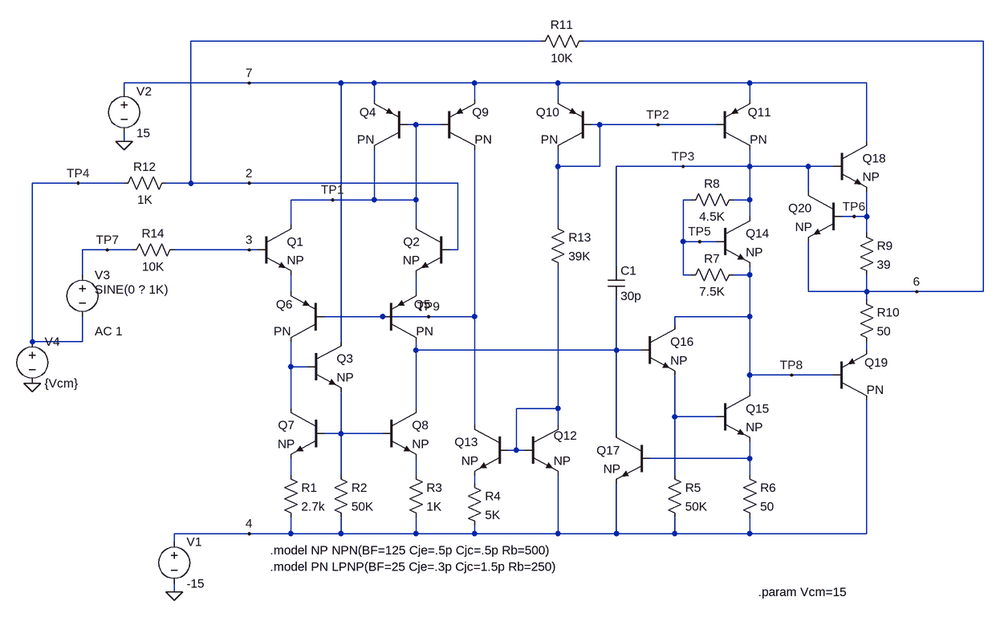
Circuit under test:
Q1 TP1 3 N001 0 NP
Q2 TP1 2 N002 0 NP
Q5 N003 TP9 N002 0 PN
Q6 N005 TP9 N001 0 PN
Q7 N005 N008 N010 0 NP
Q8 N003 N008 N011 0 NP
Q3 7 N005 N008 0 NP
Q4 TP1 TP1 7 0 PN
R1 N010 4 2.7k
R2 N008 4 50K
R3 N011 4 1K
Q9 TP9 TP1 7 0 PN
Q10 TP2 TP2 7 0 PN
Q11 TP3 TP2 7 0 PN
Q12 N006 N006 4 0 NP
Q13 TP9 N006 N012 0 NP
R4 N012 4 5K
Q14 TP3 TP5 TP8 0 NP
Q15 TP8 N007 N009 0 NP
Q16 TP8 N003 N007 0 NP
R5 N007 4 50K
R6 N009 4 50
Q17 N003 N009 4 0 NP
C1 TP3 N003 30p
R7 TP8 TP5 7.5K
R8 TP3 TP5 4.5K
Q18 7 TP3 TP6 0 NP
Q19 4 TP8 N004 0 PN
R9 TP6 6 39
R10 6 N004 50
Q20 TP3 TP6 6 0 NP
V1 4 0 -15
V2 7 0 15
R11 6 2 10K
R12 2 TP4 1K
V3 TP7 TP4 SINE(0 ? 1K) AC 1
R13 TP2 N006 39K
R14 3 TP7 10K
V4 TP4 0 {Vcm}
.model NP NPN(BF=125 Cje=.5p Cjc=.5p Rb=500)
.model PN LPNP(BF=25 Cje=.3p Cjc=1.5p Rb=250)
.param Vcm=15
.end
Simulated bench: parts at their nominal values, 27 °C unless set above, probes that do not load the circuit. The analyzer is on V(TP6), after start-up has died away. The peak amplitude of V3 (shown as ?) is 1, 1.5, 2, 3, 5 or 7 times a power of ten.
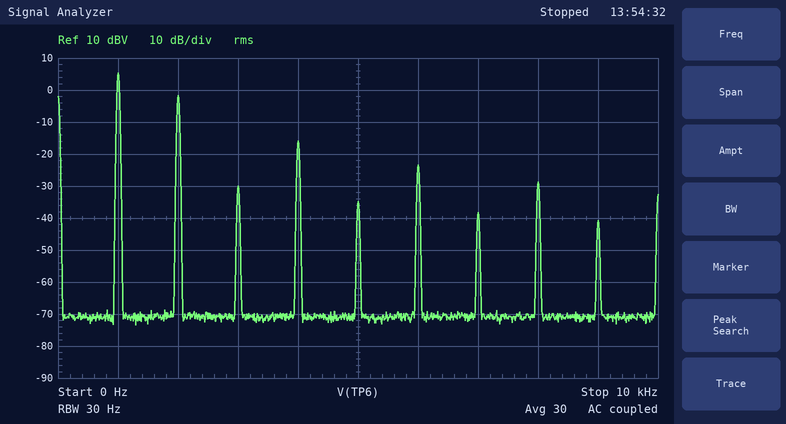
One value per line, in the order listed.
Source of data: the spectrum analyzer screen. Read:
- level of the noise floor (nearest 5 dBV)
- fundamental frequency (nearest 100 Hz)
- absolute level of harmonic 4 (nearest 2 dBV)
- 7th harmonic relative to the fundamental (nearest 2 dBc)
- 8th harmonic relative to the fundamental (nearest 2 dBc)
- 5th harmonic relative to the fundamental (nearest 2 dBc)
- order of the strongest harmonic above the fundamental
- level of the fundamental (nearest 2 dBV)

-70 dBV
1.0 kHz
-16 dBV
-44 dBc
-34 dBc
-40 dBc
2
6 dBV
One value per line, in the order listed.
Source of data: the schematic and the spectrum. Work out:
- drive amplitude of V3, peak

500 mV
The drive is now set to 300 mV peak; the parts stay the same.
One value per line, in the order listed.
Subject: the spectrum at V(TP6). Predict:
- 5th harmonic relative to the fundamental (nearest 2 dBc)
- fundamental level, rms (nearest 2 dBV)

-36 dBc
0 dBV
